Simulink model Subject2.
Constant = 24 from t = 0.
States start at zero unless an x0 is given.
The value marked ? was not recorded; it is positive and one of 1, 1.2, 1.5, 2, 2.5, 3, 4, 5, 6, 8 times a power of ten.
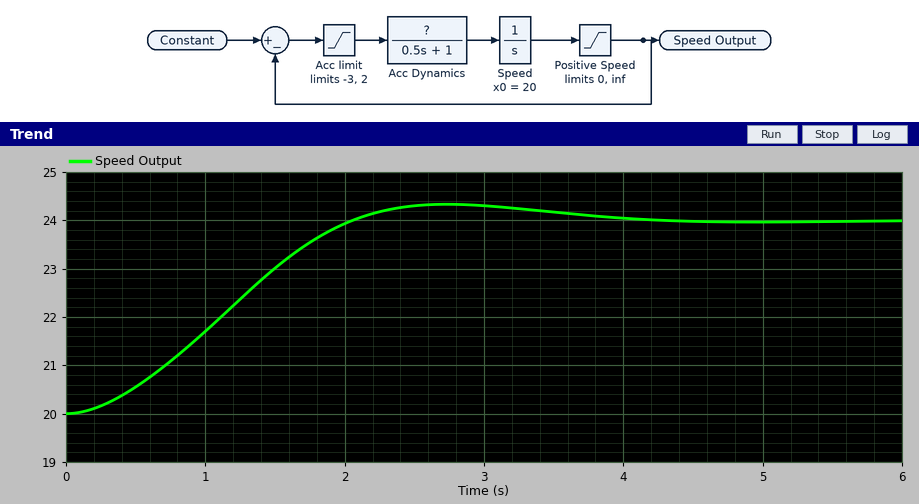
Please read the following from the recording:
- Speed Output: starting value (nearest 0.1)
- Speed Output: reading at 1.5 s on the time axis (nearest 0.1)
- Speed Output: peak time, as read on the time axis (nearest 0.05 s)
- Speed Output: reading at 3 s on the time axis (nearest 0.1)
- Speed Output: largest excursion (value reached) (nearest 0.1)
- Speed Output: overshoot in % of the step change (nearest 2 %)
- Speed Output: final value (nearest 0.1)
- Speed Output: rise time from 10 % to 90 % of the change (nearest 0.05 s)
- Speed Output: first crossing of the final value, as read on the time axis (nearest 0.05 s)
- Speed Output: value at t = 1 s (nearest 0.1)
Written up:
20.0
23.0
2.75 s
24.3
24.3
8 %
24.0
1.35 s
2.05 s
21.7
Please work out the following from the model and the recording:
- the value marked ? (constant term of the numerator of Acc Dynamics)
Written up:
1.5
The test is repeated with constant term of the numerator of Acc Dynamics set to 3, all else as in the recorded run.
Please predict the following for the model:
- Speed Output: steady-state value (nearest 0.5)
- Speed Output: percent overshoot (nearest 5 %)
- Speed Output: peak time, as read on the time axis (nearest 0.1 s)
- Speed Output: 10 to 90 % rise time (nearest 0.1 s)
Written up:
24.0
20 %
1.7 s
0.8 s
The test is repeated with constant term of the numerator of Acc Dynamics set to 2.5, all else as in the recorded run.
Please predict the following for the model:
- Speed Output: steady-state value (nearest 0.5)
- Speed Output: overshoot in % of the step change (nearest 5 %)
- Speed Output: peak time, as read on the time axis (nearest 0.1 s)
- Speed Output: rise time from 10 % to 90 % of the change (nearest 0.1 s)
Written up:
24.0
15 %
1.9 s
0.9 s
